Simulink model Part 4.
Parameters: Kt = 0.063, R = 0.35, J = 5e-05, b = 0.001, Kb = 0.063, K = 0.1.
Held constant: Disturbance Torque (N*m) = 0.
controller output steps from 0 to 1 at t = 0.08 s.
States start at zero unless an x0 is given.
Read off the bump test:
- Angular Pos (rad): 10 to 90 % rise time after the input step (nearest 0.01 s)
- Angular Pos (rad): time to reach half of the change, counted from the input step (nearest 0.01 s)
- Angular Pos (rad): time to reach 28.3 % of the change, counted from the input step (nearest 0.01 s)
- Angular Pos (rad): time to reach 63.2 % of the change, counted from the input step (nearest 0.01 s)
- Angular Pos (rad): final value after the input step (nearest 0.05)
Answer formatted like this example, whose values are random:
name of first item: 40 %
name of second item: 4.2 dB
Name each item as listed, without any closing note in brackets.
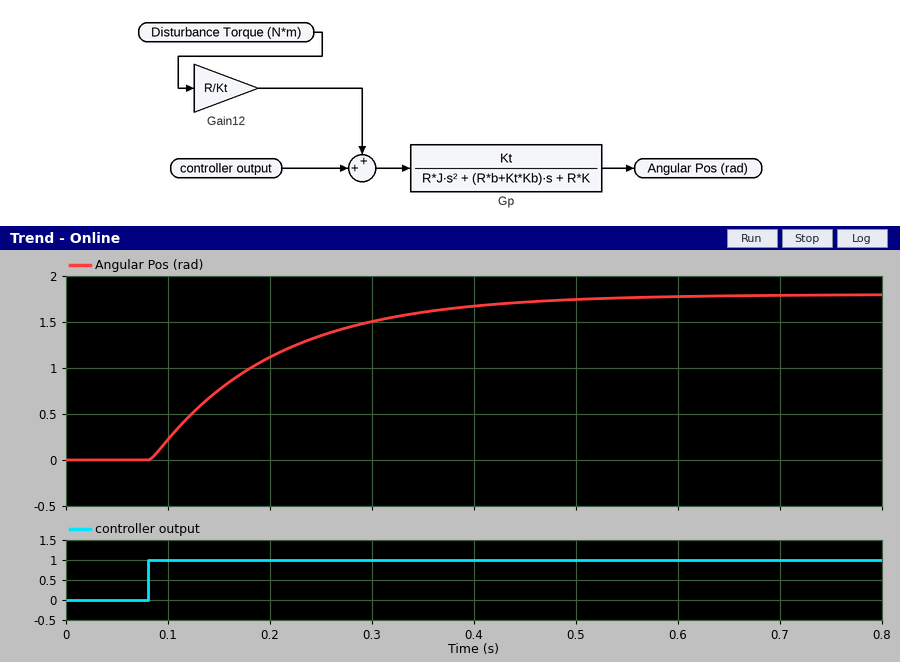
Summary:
Angular Pos (rad): 10 to 90 % rise time after the input step: 0.26 s
Angular Pos (rad): time to reach half of the change, counted from the input step: 0.09 s
Angular Pos (rad): time to reach 28.3 % of the change, counted from the input step: 0.04 s
Angular Pos (rad): time to reach 63.2 % of the change, counted from the input step: 0.12 s
Angular Pos (rad): final value after the input step: 1.80
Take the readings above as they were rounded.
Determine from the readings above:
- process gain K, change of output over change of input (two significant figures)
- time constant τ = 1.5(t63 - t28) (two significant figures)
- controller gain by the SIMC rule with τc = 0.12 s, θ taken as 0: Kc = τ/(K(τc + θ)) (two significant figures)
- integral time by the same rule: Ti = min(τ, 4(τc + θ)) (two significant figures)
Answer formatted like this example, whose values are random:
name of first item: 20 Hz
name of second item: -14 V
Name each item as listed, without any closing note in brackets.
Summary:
process gain K, change of output over change of input: 1.8
time constant τ = 1.5(t63 - t28): 0.12 s
controller gain by the SIMC rule with τc = 0.12 s, θ taken as 0: Kc = τ/(K(τc + θ)): 0.56
integral time by the same rule: Ti = min(τ, 4(τc + θ)): 0.12 s
